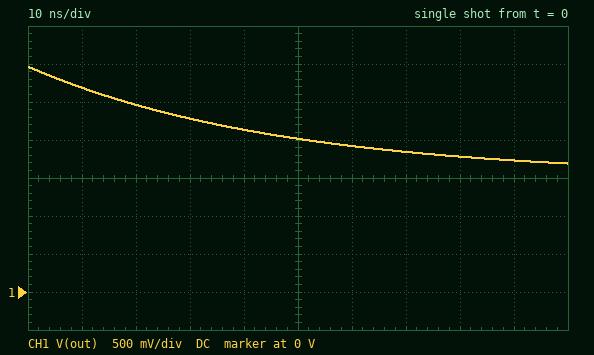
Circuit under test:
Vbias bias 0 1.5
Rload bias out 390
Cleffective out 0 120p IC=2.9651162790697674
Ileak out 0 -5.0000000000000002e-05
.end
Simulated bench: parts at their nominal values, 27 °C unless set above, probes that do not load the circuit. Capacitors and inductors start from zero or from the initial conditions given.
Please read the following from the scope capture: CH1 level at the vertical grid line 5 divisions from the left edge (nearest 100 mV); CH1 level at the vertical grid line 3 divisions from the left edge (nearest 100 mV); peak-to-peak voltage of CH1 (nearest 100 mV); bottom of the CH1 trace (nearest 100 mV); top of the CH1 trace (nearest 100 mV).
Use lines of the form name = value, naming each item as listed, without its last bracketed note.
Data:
CH1 level at the vertical grid line 5 divisions from the left edge = 2.0 V
CH1 level at the vertical grid line 3 divisions from the left edge = 2.3 V
peak-to-peak voltage of CH1 = 1.3 V
bottom of the CH1 trace = 1.7 V
top of the CH1 trace = 3.0 V
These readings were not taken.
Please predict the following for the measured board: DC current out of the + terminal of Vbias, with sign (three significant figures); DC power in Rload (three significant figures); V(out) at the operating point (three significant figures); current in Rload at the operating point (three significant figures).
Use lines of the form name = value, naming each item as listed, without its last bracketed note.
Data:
DC current out of the + terminal of Vbias, with sign = -50.0 µA
DC power in Rload = 975 nW
V(out) at the operating point = 1.52 V
current in Rload at the operating point = 50.0 µA
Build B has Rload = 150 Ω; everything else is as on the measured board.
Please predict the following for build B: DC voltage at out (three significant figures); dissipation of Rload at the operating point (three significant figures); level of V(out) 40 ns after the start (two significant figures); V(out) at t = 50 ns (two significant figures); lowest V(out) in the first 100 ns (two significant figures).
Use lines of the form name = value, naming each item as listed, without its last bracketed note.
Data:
DC voltage at out = 1.51 V
dissipation of Rload at the operating point = 375 nW
level of V(out) 40 ns after the start = 1.7 V
V(out) at t = 50 ns = 1.6 V
lowest V(out) in the first 100 ns = 1.5 V
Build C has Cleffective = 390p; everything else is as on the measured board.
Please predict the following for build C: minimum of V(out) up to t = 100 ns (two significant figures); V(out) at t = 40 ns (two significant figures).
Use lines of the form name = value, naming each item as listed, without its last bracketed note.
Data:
minimum of V(out) up to t = 100 ns = 2.3 V
V(out) at t = 40 ns = 2.6 V
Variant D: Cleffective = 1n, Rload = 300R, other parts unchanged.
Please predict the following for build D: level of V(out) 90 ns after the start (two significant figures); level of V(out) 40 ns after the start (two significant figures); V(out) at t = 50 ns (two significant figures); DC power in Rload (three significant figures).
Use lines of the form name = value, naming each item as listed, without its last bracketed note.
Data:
level of V(out) 90 ns after the start = 2.6 V
level of V(out) 40 ns after the start = 2.8 V
V(out) at t = 50 ns = 2.7 V
DC power in Rload = 750 nW
